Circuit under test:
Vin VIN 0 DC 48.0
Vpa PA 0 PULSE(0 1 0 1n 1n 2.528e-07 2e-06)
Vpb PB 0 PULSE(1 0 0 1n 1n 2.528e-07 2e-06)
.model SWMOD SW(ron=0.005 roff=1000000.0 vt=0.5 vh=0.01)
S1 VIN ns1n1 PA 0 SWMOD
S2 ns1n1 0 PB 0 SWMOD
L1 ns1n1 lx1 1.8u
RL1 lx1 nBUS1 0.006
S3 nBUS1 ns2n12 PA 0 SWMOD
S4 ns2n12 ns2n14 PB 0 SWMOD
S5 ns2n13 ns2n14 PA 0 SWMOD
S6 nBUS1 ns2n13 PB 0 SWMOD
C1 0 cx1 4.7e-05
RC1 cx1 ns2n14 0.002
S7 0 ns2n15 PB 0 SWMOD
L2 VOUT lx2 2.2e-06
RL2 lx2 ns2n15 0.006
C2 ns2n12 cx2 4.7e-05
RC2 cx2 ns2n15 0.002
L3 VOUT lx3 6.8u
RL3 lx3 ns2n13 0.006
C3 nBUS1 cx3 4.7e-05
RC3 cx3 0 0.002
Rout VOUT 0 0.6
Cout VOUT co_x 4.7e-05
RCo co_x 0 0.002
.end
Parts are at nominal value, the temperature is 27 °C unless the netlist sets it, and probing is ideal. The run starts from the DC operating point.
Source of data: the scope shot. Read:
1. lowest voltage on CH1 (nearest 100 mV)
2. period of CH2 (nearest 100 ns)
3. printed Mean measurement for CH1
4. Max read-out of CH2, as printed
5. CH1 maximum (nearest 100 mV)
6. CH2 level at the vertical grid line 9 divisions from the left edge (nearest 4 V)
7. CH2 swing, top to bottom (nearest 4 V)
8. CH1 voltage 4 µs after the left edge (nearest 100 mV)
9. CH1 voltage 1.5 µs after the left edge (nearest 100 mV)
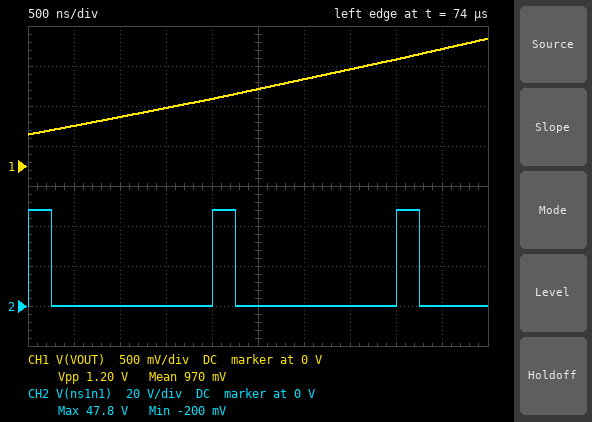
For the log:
400 mV
2.0 µs
970 mV
47.8 V
1.6 V
0 V
48 V
1.3 V
700 mV
